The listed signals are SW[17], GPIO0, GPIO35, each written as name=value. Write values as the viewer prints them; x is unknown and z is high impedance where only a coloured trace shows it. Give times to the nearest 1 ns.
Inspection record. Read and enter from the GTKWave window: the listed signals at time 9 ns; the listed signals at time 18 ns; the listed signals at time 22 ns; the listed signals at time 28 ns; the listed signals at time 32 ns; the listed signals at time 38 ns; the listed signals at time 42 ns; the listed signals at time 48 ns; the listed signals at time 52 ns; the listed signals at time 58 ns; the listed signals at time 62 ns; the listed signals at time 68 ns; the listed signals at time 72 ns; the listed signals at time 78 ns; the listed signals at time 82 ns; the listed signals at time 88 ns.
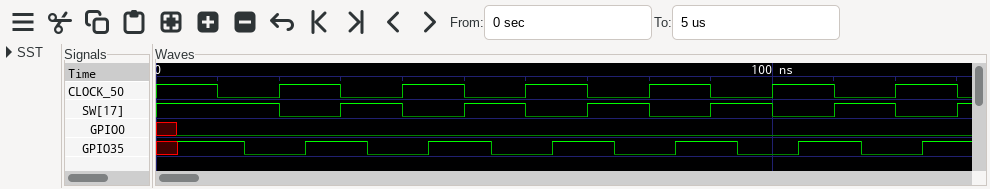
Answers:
SW[17]=1, GPIO0=0, GPIO35=1
SW[17]=1, GPIO0=0, GPIO35=0
SW[17]=0, GPIO0=0, GPIO35=0
SW[17]=0, GPIO0=0, GPIO35=1
SW[17]=1, GPIO0=0, GPIO35=1
SW[17]=1, GPIO0=0, GPIO35=0
SW[17]=0, GPIO0=0, GPIO35=0
SW[17]=0, GPIO0=0, GPIO35=1
SW[17]=1, GPIO0=0, GPIO35=1
SW[17]=1, GPIO0=0, GPIO35=0
SW[17]=0, GPIO0=0, GPIO35=0
SW[17]=0, GPIO0=0, GPIO35=1
SW[17]=1, GPIO0=0, GPIO35=1
SW[17]=1, GPIO0=0, GPIO35=0
SW[17]=0, GPIO0=0, GPIO35=0
SW[17]=0, GPIO0=0, GPIO35=1
